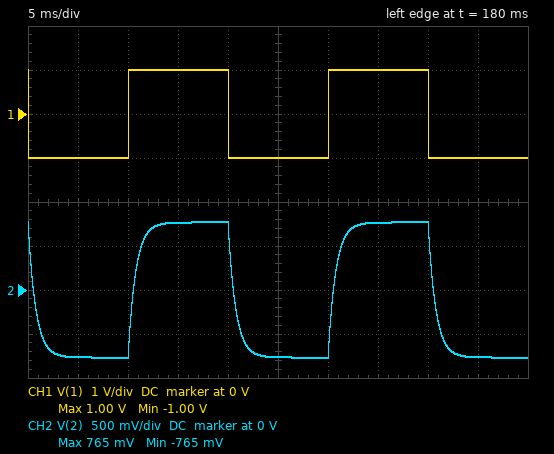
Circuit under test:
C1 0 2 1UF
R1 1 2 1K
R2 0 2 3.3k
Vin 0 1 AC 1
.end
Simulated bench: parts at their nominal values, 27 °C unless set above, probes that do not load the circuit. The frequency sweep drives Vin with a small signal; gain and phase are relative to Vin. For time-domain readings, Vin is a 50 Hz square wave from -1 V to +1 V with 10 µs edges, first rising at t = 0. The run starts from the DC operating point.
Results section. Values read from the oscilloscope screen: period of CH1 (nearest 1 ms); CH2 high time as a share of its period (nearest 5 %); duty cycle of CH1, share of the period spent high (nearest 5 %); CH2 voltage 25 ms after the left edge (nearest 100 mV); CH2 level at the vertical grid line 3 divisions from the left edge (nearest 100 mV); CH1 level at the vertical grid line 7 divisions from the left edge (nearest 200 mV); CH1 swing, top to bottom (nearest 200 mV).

20 ms
50 %
50 %
-800 mV
800 mV
1.0 V
2.0 V
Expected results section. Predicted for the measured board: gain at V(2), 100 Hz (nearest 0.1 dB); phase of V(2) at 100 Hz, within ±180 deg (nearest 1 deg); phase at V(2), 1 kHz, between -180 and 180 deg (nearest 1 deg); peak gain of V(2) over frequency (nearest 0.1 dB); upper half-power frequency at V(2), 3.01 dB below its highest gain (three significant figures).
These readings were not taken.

-3.2 dB
154 deg
102 deg
-2.3 dB
207 Hz
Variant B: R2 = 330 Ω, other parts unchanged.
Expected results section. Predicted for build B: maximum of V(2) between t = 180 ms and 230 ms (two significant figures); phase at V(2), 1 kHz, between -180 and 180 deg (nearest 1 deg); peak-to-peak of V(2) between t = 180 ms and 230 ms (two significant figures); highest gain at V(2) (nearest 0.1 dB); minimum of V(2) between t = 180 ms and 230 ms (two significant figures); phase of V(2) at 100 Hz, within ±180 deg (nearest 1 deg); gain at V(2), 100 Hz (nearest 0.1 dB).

250 mV
123 deg
500 mV
-12.1 dB
-250 mV
171 deg
-12.2 dB
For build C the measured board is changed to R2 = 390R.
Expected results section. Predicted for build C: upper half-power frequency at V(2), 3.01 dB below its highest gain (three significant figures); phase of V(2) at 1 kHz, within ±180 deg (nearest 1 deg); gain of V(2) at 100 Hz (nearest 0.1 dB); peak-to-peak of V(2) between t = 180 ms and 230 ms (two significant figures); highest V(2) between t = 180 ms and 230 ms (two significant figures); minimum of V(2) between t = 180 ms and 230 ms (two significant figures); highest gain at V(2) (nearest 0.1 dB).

567 Hz
120 deg
-11.2 dB
560 mV
280 mV
-280 mV
-11.0 dB
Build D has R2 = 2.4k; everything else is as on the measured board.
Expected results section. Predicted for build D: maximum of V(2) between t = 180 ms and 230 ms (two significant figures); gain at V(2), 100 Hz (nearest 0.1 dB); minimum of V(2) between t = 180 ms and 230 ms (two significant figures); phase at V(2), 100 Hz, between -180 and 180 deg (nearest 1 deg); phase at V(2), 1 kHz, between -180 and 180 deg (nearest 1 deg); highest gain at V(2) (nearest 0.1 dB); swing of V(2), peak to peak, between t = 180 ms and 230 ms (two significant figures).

710 mV
-3.8 dB
-710 mV
156 deg
103 deg
-3.0 dB
1.4 V
